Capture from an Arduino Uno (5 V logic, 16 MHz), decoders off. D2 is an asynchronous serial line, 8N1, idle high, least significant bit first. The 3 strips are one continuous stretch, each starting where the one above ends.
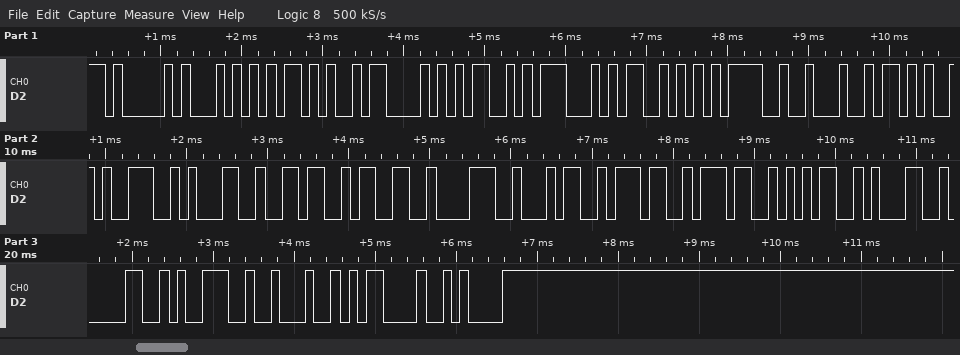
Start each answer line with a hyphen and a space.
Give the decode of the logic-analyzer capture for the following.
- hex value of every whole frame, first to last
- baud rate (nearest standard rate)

- 41 54 2B 43 4D 47 53 3D 22 2B 39 31 36 33 38 34 37 37 35 31 30 39 22 0D 0A
- 9600 baud
